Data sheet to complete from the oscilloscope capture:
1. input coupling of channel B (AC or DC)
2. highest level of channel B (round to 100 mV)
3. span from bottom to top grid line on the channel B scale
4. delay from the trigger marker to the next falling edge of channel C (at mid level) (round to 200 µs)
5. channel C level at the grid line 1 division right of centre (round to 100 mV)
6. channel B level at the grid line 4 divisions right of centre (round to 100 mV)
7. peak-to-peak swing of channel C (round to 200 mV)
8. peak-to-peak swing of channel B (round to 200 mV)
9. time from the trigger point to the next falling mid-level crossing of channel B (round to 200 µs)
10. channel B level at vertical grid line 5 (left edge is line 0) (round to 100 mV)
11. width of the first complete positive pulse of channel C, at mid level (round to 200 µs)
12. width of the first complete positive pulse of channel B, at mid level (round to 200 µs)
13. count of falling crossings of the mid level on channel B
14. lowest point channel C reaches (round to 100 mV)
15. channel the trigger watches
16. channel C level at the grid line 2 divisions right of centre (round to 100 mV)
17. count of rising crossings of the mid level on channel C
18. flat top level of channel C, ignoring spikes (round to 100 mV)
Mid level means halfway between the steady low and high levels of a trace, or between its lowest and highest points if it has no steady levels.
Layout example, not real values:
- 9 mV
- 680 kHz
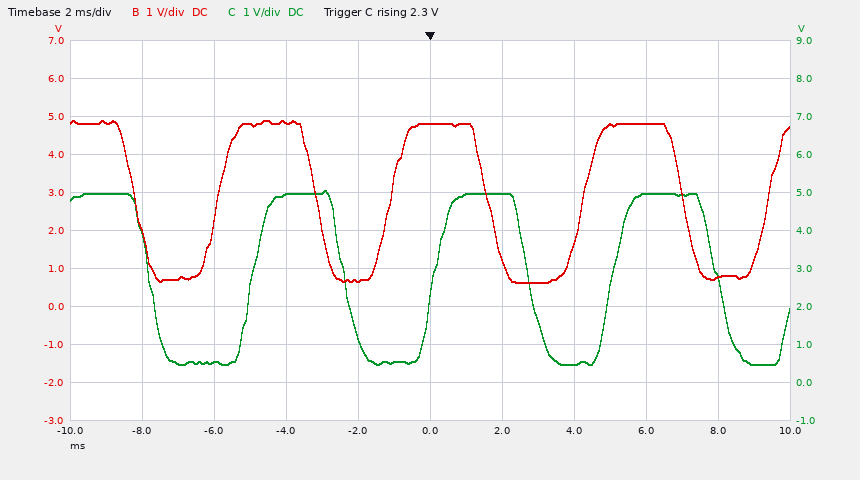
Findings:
- DC
- 4.9 V
- 10 V
- 2.8 ms
- 5.0 V
- 800 mV
- 4.6 V
- 4.2 V
- 1.6 ms
- 4.8 V
- 2.6 ms
- 2.8 ms
- 4
- 500 mV
- channel C
- 500 mV
- 3
- 5.0 V
